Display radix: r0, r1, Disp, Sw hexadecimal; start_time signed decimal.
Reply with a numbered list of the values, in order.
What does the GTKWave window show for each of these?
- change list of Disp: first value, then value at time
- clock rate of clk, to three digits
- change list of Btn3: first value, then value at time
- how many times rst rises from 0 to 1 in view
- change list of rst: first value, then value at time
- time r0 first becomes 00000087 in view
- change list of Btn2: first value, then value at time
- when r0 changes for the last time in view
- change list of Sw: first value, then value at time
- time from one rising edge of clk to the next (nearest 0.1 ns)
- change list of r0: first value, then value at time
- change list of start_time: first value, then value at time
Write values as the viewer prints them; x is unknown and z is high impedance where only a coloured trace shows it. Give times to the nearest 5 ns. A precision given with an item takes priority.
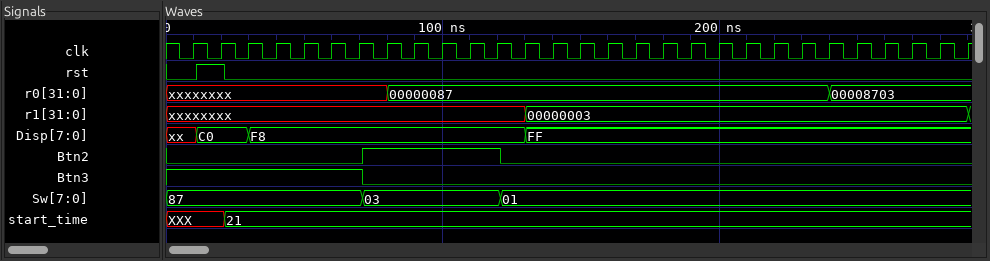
1. xx, C0 at 10 ns, F8 at 30 ns, FF at 130 ns
2. 100 MHz
3. 1, 0 at 70 ns
4. 1
5. 0, 1 at 10 ns, 0 at 20 ns
6. 80 ns
7. 0, 1 at 70 ns, 0 at 120 ns
8. 240 ns
9. 87, 03 at 70 ns, 01 at 120 ns
10. 10 ns
11. xxxxxxxx, 00000087 at 80 ns, 00008703 at 240 ns
12. XXX, 21 at 20 ns
